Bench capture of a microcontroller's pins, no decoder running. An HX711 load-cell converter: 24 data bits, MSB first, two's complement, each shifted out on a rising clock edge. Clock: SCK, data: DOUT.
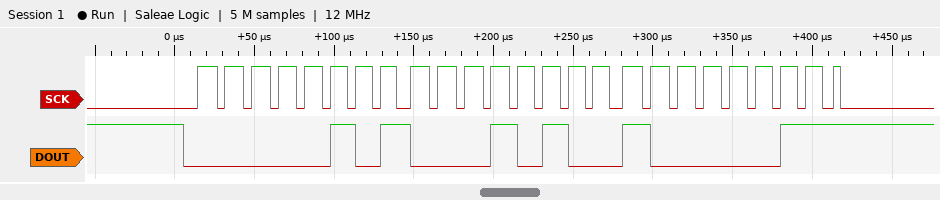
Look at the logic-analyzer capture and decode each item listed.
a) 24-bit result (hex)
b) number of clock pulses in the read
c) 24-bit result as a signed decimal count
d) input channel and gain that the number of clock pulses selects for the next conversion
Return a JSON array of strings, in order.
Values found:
["0x051483", "25", "332931", "channel A, gain 128"]
